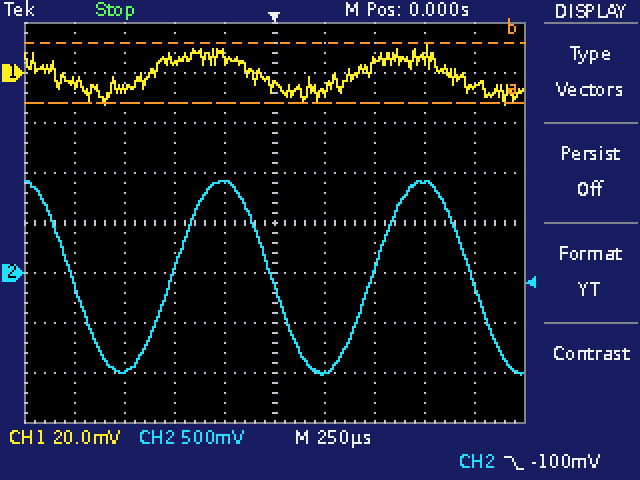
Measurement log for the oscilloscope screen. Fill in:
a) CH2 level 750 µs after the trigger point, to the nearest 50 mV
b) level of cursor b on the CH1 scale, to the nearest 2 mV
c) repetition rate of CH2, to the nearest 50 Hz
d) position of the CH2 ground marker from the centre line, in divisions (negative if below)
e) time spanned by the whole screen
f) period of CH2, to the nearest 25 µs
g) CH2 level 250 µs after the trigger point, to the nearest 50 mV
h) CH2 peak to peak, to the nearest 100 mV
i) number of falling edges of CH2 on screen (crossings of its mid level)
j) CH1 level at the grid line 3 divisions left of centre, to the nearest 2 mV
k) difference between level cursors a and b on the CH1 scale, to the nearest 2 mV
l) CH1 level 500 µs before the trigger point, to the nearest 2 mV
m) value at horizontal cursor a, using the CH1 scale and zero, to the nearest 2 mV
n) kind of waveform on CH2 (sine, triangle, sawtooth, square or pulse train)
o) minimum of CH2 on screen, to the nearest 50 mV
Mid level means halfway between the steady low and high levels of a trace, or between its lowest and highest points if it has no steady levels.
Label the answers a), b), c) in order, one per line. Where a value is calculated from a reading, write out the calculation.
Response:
a) 900 mV
b) 12 mV
c) 1 / 1.000 ms ≈ 1.00 kHz
d) -1.0 div
e) 2.5 ms
f) 1.000 ms
g) -1.00 V
h) 1.90 V
i) 3
j) -6 mV
k) 24 mV
l) 4 mV
m) -12 mV
n) sine
o) -1.00 V
